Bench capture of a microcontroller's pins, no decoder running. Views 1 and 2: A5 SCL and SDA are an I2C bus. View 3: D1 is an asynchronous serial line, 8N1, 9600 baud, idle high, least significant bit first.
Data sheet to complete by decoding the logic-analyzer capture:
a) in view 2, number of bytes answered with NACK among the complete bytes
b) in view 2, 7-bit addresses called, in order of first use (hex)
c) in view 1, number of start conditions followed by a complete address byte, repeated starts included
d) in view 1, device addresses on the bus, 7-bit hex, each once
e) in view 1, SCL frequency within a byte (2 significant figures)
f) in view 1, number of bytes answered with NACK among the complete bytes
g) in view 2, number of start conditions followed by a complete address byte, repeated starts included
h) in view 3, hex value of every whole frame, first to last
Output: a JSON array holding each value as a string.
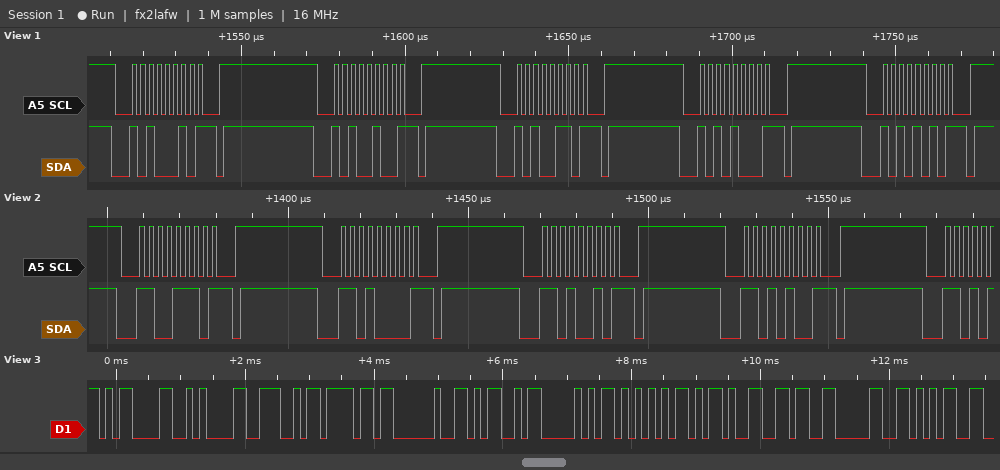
["4", "0x67 0x68 0x69 0x6A", "5", "0x51 0x52 0x53 0x54 0x55", "400 kHz", "5", "4", "0D 0A 4E 6F 20 4D 50 55 2D 36 30 35"]
